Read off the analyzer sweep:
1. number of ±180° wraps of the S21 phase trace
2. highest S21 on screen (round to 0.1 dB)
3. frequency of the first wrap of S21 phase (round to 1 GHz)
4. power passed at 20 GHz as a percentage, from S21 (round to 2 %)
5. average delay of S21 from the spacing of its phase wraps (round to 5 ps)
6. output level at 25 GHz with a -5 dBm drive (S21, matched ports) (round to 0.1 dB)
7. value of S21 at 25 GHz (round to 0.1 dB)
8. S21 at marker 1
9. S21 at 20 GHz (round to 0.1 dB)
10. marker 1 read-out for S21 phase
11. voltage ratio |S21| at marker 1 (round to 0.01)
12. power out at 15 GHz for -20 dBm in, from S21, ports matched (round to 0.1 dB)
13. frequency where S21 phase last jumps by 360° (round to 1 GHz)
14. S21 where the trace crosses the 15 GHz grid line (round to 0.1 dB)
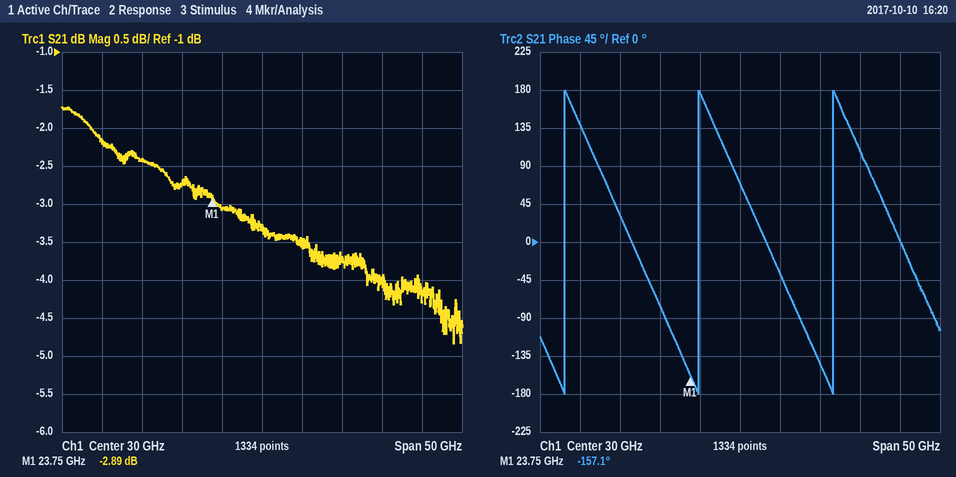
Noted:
3
-1.7 dB
8 GHz
54 %
60 ps
-8.1 dBm
-3.1 dB
-2.89 dB
-2.7 dB
-157.1°
0.72
-22.4 dBm
42 GHz
-2.4 dB
